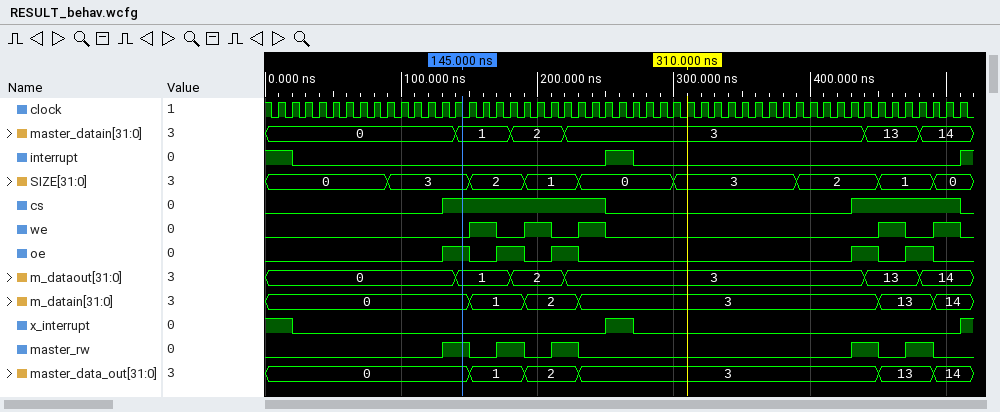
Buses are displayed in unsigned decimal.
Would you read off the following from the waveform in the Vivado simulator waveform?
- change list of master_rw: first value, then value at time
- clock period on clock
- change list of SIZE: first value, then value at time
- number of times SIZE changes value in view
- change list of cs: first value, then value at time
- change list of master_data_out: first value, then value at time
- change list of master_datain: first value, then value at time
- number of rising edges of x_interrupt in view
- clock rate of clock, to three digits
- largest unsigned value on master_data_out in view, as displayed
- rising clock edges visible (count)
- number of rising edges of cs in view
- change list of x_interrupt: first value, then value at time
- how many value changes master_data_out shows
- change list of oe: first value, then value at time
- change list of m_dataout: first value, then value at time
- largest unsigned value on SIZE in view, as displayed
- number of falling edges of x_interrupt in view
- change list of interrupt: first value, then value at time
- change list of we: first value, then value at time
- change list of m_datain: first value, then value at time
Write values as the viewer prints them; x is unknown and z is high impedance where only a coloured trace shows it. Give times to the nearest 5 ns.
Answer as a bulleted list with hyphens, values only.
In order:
- 0, 1 at 130 ns, 0 at 150 ns, 1 at 170 ns, 0 at 190 ns, 1 at 210 ns, 0 at 230 ns, 1 at 430 ns, 0 at 450 ns, 1 at 470 ns, 0 at 490 ns
- 10 ns
- 0, 3 at 90 ns, 2 at 150 ns, 1 at 190 ns, 0 at 230 ns, 3 at 300 ns, 2 at 390 ns, 1 at 450 ns, 0 at 490 ns
- 8
- 0, 1 at 130 ns, 0 at 250 ns, 1 at 430 ns, 0 at 510 ns
- 0, 1 at 150 ns, 2 at 190 ns, 3 at 230 ns, 13 at 450 ns, 14 at 490 ns
- 0, 1 at 140 ns, 2 at 180 ns, 3 at 220 ns, 13 at 440 ns, 14 at 480 ns
- 2
- 100 MHz
- 14
- 51
- 2
- 1, 0 at 20 ns, 1 at 250 ns, 0 at 270 ns, 1 at 510 ns
- 5
- 0, 1 at 130 ns, 0 at 150 ns, 1 at 170 ns, 0 at 190 ns, 1 at 210 ns, 0 at 230 ns, 1 at 430 ns, 0 at 450 ns, 1 at 470 ns, 0 at 490 ns
- 0, 1 at 140 ns, 2 at 180 ns, 3 at 220 ns, 13 at 440 ns, 14 at 480 ns
- 3
- 2
- 1, 0 at 20 ns, 1 at 250 ns, 0 at 270 ns, 1 at 510 ns
- 0, 1 at 150 ns, 0 at 170 ns, 1 at 190 ns, 0 at 210 ns, 1 at 230 ns, 0 at 250 ns, 1 at 450 ns, 0 at 470 ns, 1 at 490 ns, 0 at 510 ns
- 0, 1 at 150 ns, 2 at 190 ns, 3 at 230 ns, 13 at 450 ns, 14 at 490 ns
